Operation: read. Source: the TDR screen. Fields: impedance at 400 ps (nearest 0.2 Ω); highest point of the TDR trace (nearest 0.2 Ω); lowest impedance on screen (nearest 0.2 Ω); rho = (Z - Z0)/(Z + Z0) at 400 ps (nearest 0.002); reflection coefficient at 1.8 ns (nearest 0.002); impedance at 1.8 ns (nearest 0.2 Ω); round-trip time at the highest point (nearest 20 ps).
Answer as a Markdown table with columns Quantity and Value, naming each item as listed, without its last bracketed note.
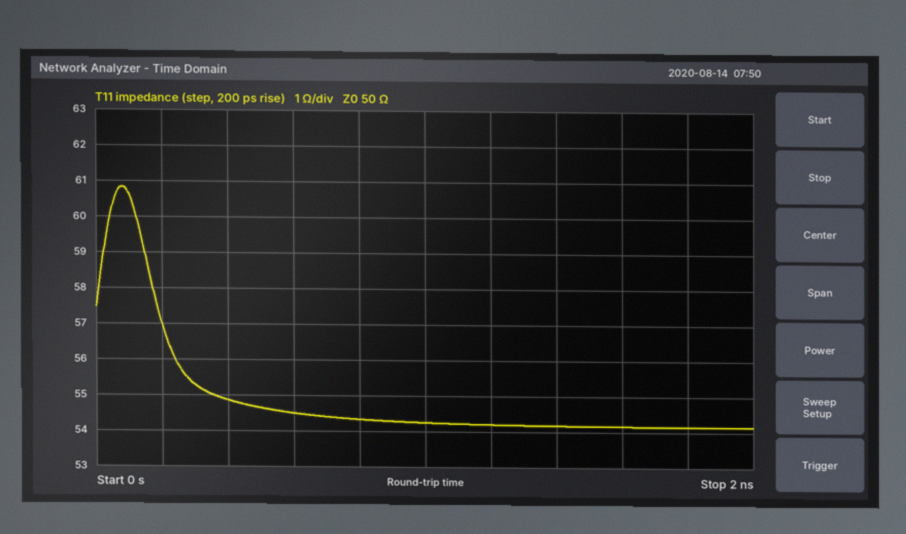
| Quantity | Value |
|---|---|
| impedance at 400 ps | 54.8 Ω |
| highest point of the TDR trace | 60.8 Ω |
| lowest impedance on screen | 54.2 Ω |
| rho = (Z - Z0)/(Z + Z0) at 400 ps | +0.046 |
| reflection coefficient at 1.8 ns | +0.040 |
| impedance at 1.8 ns | 54.2 Ω |
| round-trip time at the highest point | 80 ps |
